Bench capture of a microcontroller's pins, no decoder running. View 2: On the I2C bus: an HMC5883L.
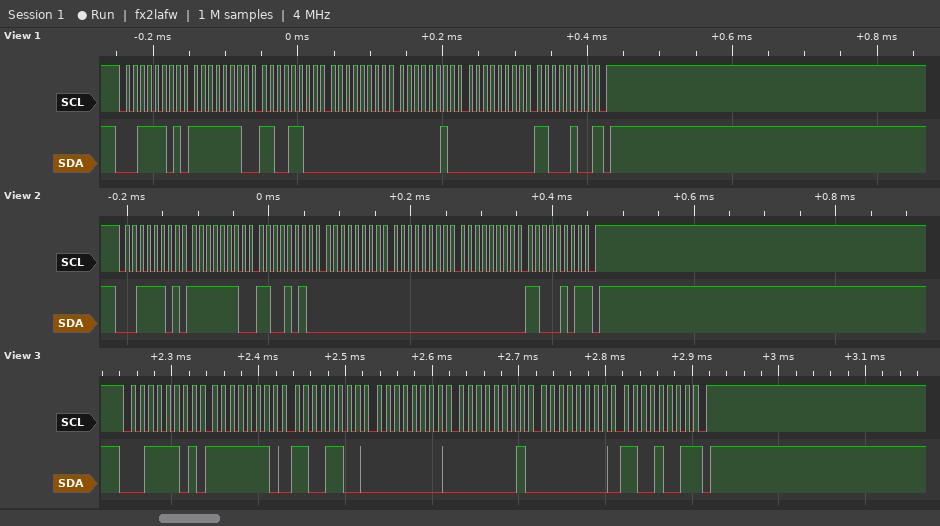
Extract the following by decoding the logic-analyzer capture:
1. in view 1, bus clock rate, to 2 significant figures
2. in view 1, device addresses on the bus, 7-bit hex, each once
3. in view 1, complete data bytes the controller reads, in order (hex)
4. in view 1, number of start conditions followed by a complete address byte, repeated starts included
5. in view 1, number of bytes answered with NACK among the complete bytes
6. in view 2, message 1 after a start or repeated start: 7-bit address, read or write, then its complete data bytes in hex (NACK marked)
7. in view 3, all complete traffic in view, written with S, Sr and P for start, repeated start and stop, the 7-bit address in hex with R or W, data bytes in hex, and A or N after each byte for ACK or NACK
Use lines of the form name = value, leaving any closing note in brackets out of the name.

in view 1, bus clock rate, to 2 significant figures = 100 kHz
in view 1, device addresses on the bus, 7-bit hex, each once = 0x1E
in view 1, complete data bytes the controller reads, in order = FE CC 00 02 00 C4
in view 1, number of start conditions followed by a complete address byte, repeated starts included = 1
in view 1, number of bytes answered with NACK among the complete bytes = 1
in view 2, message 1 after a start or repeated start: 7-bit address, read or write, then its complete data bytes in hex = 0x1E read: FE CA 00 00 00 C5 NACK
in view 3, all complete traffic in view, written with S, Sr and P for start, repeated start and stop, the 7-bit address in hex with R or W, data bytes in hex, and A or N after each byte for ACK or NACK = S 1ER A FE A CC A 00 A 01 A 00 A C9 N P
